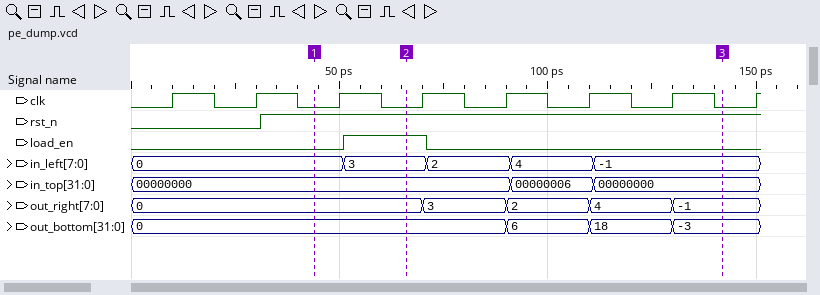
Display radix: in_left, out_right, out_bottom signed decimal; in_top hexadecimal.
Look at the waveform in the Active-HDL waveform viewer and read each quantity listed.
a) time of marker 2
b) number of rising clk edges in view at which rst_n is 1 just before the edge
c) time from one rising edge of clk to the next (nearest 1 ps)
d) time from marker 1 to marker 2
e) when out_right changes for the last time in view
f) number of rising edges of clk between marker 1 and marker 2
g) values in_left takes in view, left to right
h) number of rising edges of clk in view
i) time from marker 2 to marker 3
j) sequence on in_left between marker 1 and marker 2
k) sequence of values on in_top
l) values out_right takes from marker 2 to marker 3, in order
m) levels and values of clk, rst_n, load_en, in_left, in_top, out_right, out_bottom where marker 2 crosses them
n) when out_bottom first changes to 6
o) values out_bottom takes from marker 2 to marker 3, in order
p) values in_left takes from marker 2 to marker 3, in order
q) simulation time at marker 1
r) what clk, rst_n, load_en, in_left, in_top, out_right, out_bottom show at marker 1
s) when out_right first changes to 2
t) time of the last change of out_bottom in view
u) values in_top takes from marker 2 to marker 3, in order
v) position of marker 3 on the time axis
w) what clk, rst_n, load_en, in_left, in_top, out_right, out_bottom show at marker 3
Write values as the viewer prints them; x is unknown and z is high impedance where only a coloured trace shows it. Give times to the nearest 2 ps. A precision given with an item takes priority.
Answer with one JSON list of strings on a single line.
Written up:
["66 ps", "6", "20 ps", "22 ps", "130 ps", "1", "0, 3, 2, 4, -1", "8", "76 ps", "0, 3", "00000000, 00000006, 00000000", "0, 3, 2, 4, -1", "clk=0, rst_n=1, load_en=1, in_left=3, in_top=00000000, out_right=0, out_bottom=0", "90 ps", "0, 6, 18, -3", "3, 2, 4, -1", "44 ps", "clk=0, rst_n=1, load_en=0, in_left=0, in_top=00000000, out_right=0, out_bottom=0", "90 ps", "130 ps", "00000000, 00000006, 00000000", "142 ps", "clk=0, rst_n=1, load_en=0, in_left=-1, in_top=00000000, out_right=-1, out_bottom=-3"]
